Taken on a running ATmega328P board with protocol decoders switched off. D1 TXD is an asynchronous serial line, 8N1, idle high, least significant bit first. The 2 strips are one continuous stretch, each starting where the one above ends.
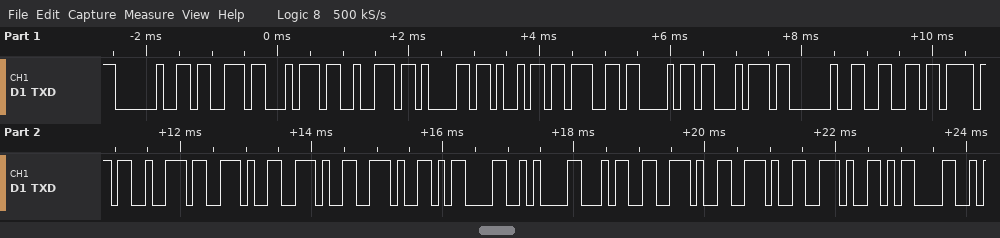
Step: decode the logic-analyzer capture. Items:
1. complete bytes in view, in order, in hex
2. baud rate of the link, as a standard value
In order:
0x20 0x73 0x74 0x72 0x61 0x69 0x67 0x68 0x74 0x20 0x66 0x6F 0x72 0x2E 0x2E 0x2E 0x0D 0x0A 0x34 0x2E 0x2E 0x2E 0x0D
9600 baud
